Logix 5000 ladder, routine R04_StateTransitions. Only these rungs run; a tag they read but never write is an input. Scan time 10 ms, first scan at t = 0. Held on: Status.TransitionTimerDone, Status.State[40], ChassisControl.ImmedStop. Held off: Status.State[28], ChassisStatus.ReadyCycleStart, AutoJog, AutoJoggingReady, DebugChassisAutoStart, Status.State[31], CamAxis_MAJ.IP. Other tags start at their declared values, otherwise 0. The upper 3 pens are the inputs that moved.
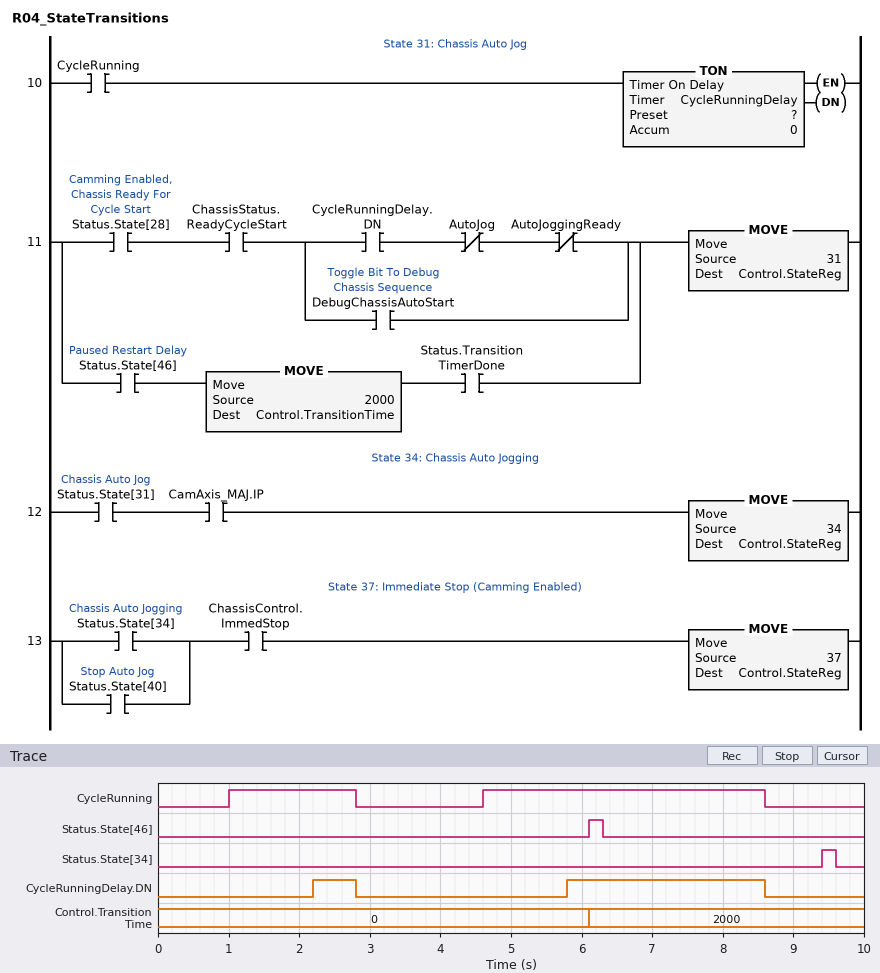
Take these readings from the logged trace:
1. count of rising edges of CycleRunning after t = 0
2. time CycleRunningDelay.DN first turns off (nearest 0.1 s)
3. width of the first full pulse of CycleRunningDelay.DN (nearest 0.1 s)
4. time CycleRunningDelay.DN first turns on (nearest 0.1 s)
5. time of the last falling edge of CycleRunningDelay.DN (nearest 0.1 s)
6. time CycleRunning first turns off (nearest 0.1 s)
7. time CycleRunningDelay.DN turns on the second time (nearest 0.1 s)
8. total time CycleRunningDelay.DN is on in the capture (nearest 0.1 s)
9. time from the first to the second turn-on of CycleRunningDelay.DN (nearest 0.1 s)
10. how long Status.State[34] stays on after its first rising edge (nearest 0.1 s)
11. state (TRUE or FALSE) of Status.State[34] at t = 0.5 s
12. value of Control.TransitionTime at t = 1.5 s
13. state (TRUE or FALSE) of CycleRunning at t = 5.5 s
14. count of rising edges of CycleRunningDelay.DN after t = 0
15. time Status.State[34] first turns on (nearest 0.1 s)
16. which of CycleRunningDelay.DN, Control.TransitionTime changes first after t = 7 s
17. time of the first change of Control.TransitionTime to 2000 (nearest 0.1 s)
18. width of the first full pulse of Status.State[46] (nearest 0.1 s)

2
2.8 s
0.6 s
2.2 s
8.6 s
2.8 s
5.8 s
3.4 s
3.6 s
0.2 s
FALSE
0
TRUE
2
9.4 s
CycleRunningDelay.DN
6.1 s
0.2 s
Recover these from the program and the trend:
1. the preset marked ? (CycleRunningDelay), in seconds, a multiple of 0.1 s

1.2 s
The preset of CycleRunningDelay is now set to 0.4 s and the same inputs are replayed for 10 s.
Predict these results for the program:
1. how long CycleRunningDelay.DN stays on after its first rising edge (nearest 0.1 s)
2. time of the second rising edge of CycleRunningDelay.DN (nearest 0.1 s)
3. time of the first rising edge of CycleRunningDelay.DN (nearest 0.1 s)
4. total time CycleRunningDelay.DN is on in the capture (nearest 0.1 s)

1.4 s
5.0 s
1.4 s
5.0 s
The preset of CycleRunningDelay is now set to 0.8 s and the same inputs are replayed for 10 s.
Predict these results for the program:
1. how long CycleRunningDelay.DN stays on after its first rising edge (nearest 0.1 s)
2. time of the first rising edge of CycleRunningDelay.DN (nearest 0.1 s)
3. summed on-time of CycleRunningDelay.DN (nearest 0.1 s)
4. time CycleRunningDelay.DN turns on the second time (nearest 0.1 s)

1.0 s
1.8 s
4.2 s
5.4 s
